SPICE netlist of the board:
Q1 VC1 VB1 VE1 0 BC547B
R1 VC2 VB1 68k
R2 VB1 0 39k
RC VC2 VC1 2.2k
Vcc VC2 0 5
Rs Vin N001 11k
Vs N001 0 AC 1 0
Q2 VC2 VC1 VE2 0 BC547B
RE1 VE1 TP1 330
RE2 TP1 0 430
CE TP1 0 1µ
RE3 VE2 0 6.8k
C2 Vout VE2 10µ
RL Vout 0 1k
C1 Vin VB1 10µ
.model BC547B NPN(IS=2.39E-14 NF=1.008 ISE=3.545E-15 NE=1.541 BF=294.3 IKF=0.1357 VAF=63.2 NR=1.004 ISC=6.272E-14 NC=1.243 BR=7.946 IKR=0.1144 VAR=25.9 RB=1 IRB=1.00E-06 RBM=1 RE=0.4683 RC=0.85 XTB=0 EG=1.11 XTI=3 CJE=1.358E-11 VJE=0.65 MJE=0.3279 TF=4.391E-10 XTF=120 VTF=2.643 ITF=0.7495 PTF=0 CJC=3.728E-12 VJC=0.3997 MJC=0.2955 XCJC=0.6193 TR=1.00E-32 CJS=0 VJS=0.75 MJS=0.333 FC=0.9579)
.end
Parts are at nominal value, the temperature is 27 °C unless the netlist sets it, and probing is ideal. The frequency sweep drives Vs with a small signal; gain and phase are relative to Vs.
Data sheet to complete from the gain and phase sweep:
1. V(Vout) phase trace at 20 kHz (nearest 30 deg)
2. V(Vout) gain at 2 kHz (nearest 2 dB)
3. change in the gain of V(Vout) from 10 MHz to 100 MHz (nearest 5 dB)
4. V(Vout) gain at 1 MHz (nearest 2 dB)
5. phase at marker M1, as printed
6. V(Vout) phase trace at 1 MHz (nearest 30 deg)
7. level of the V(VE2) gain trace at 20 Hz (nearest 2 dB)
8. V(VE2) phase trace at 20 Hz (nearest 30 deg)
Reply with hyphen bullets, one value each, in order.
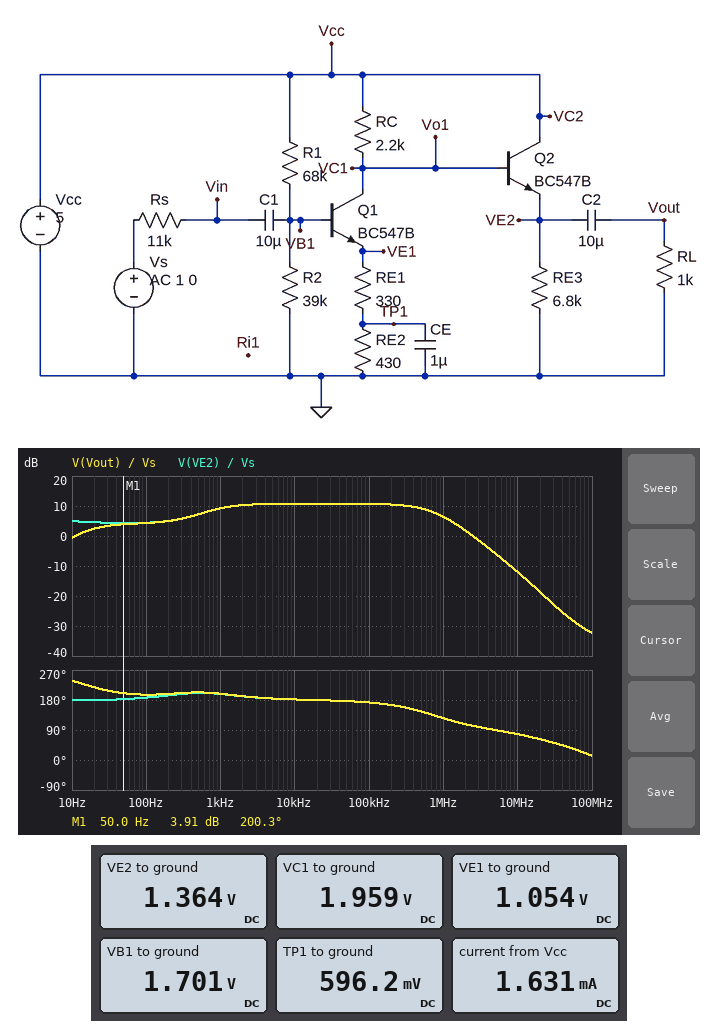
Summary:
- 180 deg
- 10 dB
- -20 dB
- 6 dB
- 200.3 deg
- 120 deg
- 4 dB
- 180 deg
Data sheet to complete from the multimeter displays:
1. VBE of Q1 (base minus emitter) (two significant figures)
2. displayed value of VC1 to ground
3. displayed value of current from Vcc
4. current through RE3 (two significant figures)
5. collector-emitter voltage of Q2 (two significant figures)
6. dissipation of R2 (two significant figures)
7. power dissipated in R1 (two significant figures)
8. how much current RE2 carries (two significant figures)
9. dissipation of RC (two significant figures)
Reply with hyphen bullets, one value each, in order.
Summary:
- 650 mV
- 1.959 V
- 1.631 mA
- 200 µA
- 3.6 V
- 74 µW
- 160 µW
- 1.4 mA
- 4.2 mW
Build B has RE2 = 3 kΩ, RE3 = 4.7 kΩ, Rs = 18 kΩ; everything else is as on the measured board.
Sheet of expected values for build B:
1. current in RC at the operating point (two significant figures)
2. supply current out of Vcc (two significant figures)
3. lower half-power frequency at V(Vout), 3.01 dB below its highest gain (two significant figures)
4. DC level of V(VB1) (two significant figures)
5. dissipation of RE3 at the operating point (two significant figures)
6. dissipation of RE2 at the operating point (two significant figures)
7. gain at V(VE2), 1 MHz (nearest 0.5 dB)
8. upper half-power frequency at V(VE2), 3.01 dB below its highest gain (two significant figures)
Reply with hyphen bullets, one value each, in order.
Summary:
- 360 µA
- 1.2 mA
- 410 Hz
- 1.8 V
- 2.7 mW
- 380 µW
- 4.5 dB
- 760 kHz
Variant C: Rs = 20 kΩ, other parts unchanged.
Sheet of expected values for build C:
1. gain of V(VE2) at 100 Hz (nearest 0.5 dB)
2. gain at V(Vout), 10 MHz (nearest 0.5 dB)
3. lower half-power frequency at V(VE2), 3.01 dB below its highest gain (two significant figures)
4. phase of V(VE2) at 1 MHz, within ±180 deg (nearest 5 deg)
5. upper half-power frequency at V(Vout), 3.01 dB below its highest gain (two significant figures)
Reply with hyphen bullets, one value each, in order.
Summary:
- 2.5 dB
- -17.0 dB
- 570 Hz
- 115 deg
- 550 kHz
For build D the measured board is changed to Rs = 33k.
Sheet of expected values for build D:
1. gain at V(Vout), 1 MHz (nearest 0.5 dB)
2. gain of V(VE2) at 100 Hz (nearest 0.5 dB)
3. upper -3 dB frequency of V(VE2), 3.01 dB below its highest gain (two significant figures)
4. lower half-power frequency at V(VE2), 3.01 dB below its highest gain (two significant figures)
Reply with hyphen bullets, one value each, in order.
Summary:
- -1.5 dB
- 0 dB
- 450 kHz
- 560 Hz
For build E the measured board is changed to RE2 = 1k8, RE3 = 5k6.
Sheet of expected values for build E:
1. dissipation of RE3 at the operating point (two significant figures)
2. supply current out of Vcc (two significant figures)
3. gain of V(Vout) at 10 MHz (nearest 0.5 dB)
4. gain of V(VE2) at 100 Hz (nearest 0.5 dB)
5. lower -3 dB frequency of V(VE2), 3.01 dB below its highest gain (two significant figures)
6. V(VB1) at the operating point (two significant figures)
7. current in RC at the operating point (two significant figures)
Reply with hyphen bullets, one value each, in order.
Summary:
- 1.8 mW
- 1.2 mA
- -9.5 dB
- -0.5 dB
- 460 Hz
- 1.8 V
- 540 µA
